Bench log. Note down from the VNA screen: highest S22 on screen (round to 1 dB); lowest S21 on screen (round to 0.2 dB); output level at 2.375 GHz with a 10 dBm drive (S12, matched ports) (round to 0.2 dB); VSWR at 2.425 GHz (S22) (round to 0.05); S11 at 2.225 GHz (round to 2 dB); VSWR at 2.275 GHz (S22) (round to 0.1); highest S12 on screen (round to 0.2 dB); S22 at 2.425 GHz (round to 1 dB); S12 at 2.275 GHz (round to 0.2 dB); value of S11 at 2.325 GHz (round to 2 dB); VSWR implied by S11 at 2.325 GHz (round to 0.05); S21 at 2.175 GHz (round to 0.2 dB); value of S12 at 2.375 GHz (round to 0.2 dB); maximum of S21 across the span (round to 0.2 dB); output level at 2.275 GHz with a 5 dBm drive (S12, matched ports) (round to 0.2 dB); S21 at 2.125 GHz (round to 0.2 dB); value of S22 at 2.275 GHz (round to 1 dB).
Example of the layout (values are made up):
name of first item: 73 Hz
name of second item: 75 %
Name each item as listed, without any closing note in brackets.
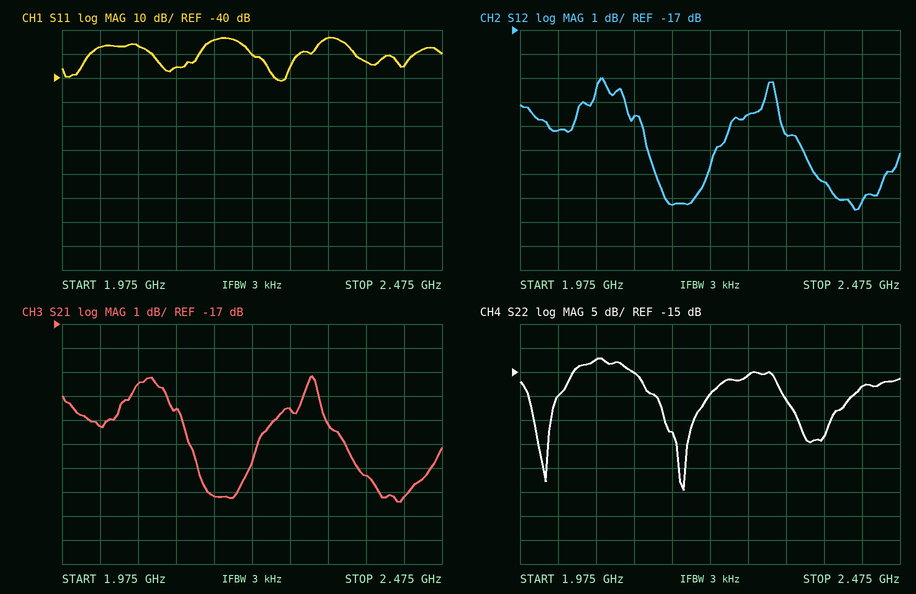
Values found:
highest S22 on screen: -12 dB
lowest S21 on screen: -24.4 dB
output level at 2.375 GHz with a 10 dBm drive (S12, matched ports): -13.4 dBm
VSWR at 2.425 GHz (S22): 1.30
S11 at 2.225 GHz: -30 dB
VSWR at 2.275 GHz (S22): 1.4
highest S12 on screen: -19.0 dB
S22 at 2.425 GHz: -18 dB
S12 at 2.275 GHz: -20.6 dB
value of S11 at 2.325 GHz: -24 dB
VSWR implied by S11 at 2.325 GHz: 1.15
S21 at 2.175 GHz: -24.2 dB
value of S12 at 2.375 GHz: -23.4 dB
maximum of S21 across the span: -19.2 dB
output level at 2.275 GHz with a 5 dBm drive (S12, matched ports): -15.6 dBm
S21 at 2.125 GHz: -20.6 dB
value of S22 at 2.275 GHz: -16 dB
